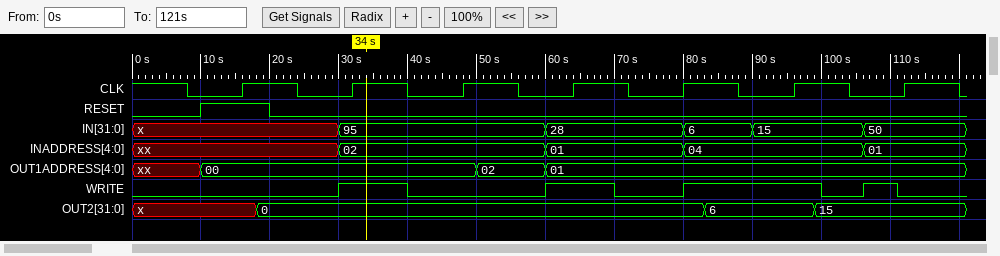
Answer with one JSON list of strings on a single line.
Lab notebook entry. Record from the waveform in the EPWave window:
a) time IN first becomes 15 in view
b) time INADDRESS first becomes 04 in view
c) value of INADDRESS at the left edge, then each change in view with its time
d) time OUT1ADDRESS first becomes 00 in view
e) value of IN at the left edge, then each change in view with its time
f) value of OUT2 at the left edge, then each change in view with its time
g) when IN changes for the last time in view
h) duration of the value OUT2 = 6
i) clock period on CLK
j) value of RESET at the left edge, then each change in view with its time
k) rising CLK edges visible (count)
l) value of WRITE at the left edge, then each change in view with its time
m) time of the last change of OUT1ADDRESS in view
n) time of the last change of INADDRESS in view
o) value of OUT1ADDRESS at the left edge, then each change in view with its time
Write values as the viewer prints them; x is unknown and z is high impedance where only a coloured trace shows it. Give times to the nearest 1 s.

["90 s", "80 s", "xx, 02 at 30 s, 01 at 60 s, 04 at 80 s, 01 at 106 s", "10 s", "x, 95 at 30 s, 28 at 60 s, 6 at 80 s, 15 at 90 s, 50 at 106 s", "x, 0 at 18 s, 6 at 83 s, 15 at 99 s", "106 s", "16 s", "16 s", "0, 1 at 10 s, 0 at 20 s", "7", "0, 1 at 30 s, 0 at 40 s, 1 at 60 s, 0 at 70 s, 1 at 80 s, 0 at 100 s, 1 at 106 s, 0 at 111 s", "60 s", "106 s", "xx, 00 at 10 s, 02 at 50 s, 01 at 60 s"]
